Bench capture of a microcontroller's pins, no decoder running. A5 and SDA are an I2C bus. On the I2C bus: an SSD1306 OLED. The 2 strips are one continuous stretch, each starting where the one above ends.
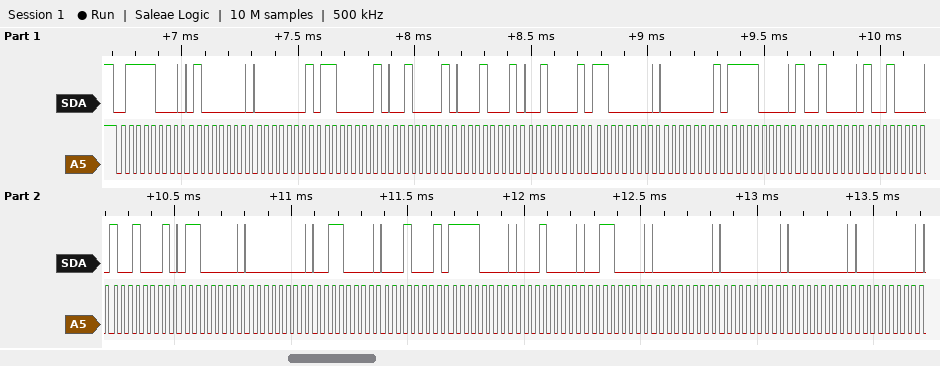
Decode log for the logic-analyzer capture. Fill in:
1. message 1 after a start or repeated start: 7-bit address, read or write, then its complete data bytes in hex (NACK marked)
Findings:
0x3C write: 40 01 C1 21 11 21 C0 01 F0 90 90 91 60 00 30 11 F0 10 30 00 00 00 00
